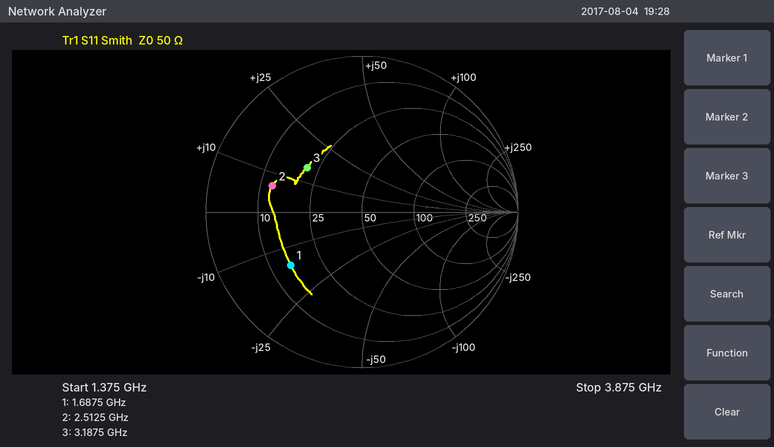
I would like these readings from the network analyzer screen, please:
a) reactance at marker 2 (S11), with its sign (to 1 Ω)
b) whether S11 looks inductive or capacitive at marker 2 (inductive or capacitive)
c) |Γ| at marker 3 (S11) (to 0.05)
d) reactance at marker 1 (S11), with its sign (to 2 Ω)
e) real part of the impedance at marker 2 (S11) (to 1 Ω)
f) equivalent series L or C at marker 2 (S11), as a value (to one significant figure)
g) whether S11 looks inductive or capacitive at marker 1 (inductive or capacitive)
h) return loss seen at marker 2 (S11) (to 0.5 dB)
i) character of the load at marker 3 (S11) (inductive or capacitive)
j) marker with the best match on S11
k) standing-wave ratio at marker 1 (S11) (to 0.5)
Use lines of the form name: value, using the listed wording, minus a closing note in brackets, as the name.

reactance at marker 2 (S11), with its sign: +7 Ω
whether S11 looks inductive or capacitive at marker 2: inductive
|Γ| at marker 3 (S11): 0.45
reactance at marker 1 (S11), with its sign: -16 Ω
real part of the impedance at marker 2 (S11): 13 Ω
equivalent series L or C at marker 2 (S11), as a value: 400 pH
whether S11 looks inductive or capacitive at marker 1: capacitive
return loss seen at marker 2 (S11): 4.5 dB
character of the load at marker 3 (S11): inductive
marker with the best match on S11: marker 3
standing-wave ratio at marker 1 (S11): 3.5
